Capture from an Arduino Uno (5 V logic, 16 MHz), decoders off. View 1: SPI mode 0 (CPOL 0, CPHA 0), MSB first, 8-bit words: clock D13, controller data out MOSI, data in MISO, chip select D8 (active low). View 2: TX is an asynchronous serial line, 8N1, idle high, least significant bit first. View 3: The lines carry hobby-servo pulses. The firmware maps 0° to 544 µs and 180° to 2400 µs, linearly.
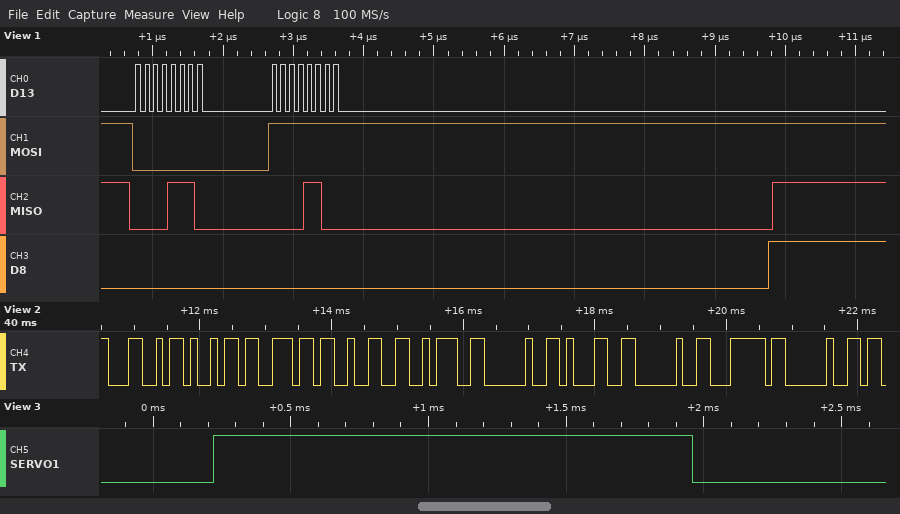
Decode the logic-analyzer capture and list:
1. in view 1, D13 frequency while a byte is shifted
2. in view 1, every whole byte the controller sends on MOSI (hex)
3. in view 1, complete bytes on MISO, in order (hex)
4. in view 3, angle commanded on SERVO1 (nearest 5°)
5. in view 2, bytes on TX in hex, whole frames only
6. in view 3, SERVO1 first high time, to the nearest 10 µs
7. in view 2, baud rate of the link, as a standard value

8 MHz
00 FF
0E 0C
115°
0x4C 0x69 0x6E 0x32 0x3A 0x20 0x31 0x20 0x7C 0x20
1740 µs
9600 baud
